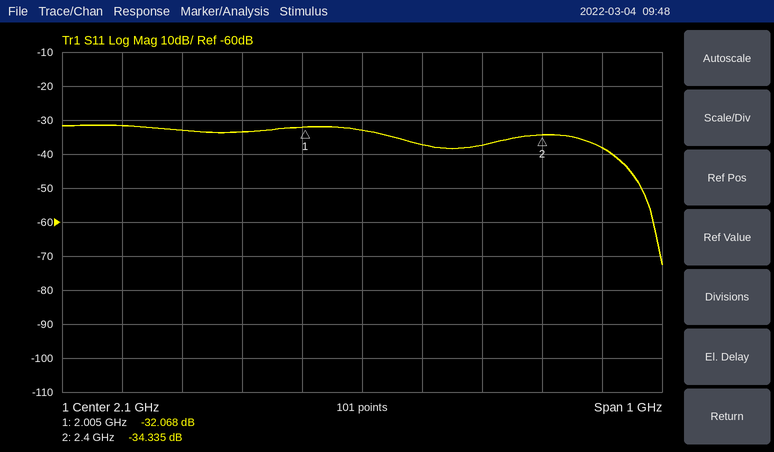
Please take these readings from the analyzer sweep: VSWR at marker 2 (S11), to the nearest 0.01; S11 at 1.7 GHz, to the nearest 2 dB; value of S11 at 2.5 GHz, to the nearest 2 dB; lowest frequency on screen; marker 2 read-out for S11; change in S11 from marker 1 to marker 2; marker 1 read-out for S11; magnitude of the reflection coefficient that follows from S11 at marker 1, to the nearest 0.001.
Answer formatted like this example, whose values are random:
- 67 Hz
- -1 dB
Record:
- 1.04
- -32 dB
- -38 dB
- 1.6 GHz
- -34.335 dB
- -2.267 dB
- -32.068 dB
- 0.025
